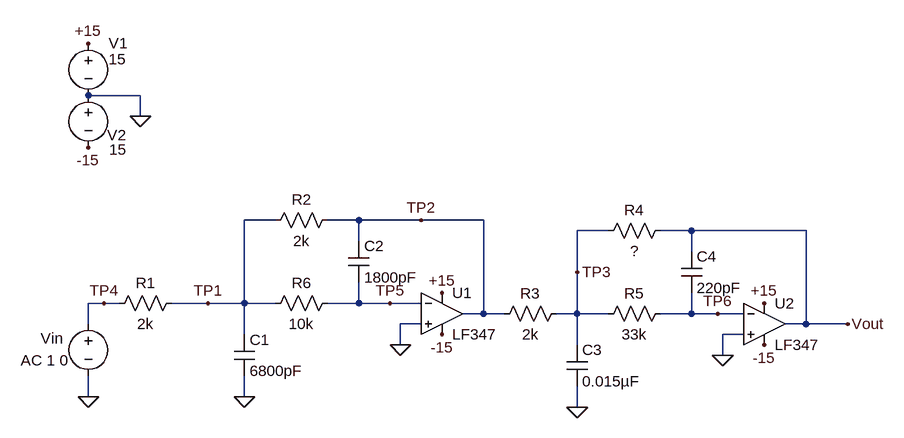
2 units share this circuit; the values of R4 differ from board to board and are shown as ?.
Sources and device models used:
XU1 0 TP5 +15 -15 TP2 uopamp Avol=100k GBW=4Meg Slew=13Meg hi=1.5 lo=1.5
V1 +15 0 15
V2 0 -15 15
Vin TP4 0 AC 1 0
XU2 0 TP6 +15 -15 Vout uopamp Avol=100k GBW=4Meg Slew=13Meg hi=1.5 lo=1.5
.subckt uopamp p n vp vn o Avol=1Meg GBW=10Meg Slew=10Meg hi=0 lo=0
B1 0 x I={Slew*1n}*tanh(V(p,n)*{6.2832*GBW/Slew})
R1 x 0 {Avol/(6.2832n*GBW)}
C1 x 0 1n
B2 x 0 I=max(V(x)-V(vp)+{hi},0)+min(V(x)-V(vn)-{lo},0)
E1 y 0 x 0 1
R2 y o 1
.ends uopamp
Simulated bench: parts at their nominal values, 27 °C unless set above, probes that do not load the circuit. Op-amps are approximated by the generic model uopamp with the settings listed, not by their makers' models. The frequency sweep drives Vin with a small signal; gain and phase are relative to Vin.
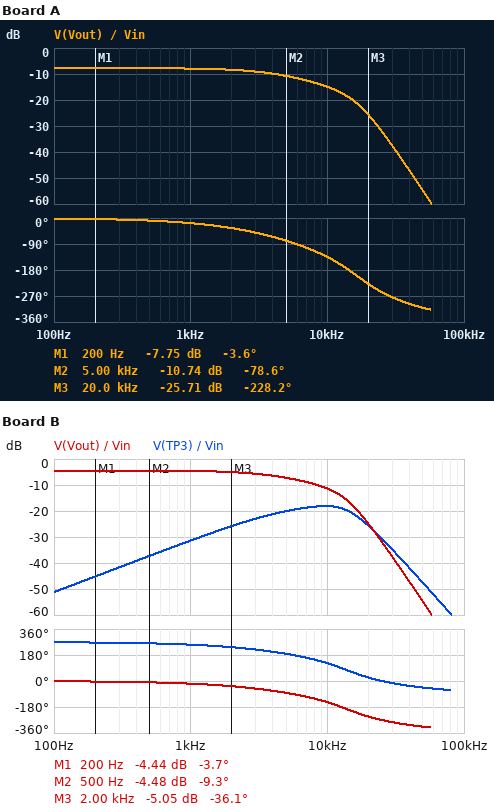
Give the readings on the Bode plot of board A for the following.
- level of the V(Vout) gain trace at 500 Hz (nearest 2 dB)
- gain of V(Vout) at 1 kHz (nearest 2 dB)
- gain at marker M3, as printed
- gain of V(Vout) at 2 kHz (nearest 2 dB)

-8 dB
-8 dB
-25.71 dB
-8 dB
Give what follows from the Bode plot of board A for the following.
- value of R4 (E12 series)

820 Ω
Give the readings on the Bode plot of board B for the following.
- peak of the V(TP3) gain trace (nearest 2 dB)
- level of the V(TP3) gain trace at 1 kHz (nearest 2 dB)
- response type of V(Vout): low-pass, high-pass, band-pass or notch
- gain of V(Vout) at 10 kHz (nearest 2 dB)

-18 dB
-32 dB
low-pass
-12 dB
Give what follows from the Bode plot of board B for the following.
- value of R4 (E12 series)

1.2 kΩ
